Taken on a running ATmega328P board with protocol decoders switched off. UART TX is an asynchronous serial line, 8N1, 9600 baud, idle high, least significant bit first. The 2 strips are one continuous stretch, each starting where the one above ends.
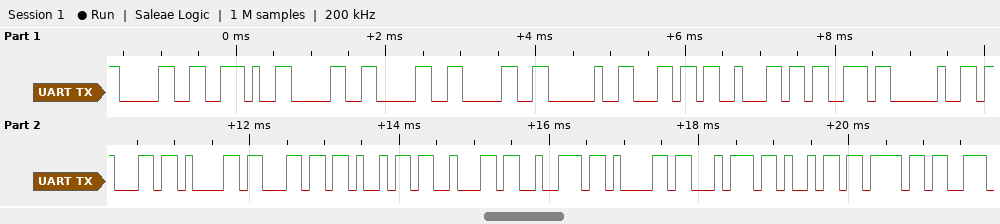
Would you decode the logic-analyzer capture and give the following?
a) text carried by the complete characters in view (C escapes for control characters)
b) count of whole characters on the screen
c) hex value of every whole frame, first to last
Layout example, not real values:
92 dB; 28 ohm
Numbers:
"0.000 lbs calibratio"; 20; 30 2E 30 30 30 20 6C 62 73 20 63 61 6C 69 62 72 61 74 69 6F
